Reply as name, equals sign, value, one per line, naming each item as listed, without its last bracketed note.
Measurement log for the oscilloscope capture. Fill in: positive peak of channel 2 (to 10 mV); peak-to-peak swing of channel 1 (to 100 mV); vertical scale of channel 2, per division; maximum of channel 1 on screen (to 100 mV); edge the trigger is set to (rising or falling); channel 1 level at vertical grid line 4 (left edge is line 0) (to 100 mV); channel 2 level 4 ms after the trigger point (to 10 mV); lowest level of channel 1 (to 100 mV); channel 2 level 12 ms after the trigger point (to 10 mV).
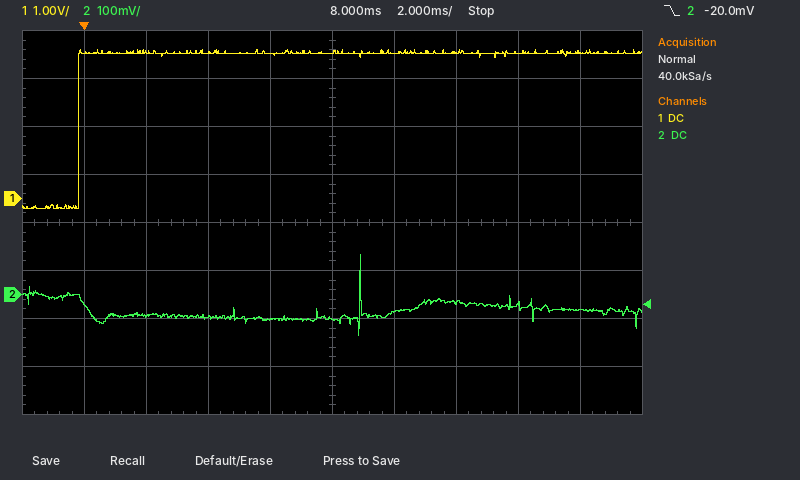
positive peak of channel 2 = 80 mV
peak-to-peak swing of channel 1 = 3.3 V
vertical scale of channel 2, per division = 100 mV
maximum of channel 1 on screen = 3.1 V
edge the trigger is set to = falling
channel 1 level at vertical grid line 4 (left edge is line 0) = 3.0 V
channel 2 level 4 ms after the trigger point = -50 mV
lowest level of channel 1 = -200 mV
channel 2 level 12 ms after the trigger point = -20 mV
